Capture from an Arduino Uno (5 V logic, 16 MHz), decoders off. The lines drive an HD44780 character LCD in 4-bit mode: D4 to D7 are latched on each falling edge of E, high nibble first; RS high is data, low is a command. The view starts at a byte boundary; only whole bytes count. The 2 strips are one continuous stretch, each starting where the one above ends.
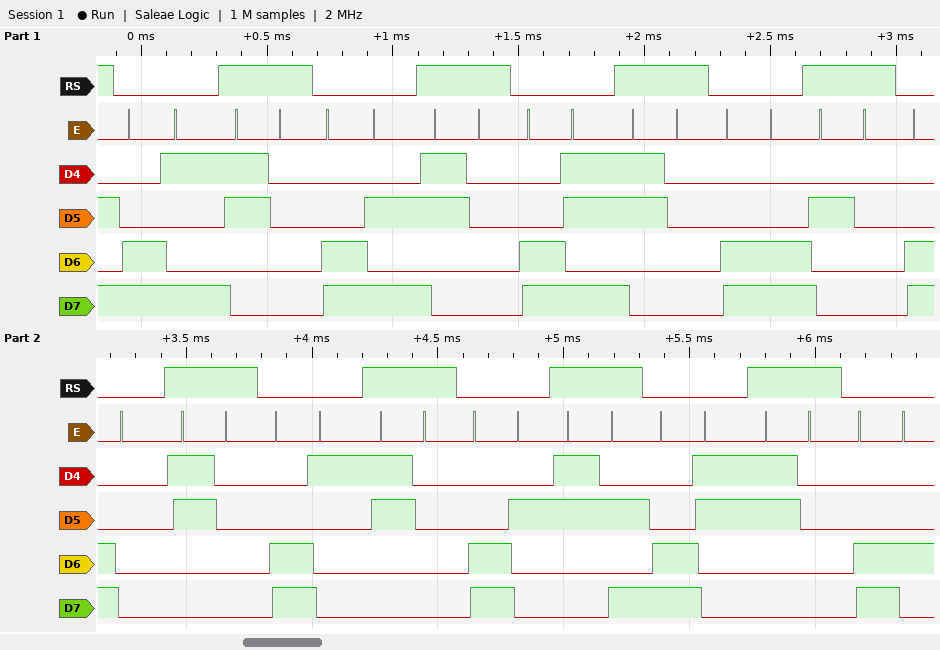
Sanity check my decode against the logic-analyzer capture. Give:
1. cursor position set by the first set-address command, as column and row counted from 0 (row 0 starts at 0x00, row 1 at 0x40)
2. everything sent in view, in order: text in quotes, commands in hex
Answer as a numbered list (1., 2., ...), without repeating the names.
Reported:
1. column 9, row 1
2. 0xC9 "0" 0xCA "0" 0xCB "0" 0xCC " " 0xC0 "0" 0xC1 "0" 0xC2 ":" 0xC3 "0" 0xC4
